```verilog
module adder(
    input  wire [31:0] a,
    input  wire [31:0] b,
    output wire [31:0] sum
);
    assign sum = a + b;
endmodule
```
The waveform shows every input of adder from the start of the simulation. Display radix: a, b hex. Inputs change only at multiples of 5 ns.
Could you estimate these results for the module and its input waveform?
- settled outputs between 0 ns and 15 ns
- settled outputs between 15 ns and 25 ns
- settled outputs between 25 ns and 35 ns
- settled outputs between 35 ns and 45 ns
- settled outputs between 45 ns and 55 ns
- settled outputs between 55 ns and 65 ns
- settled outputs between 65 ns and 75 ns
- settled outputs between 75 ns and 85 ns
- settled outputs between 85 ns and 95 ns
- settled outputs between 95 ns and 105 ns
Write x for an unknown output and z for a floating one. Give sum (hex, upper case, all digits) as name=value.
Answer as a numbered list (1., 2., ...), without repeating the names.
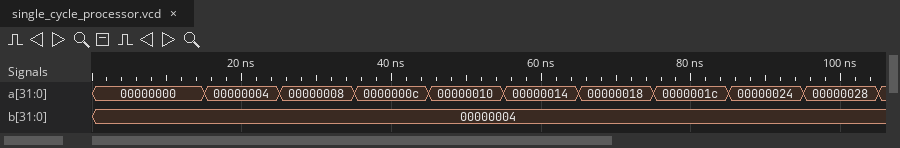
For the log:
1. sum=00000004
2. sum=00000008
3. sum=0000000C
4. sum=00000010
5. sum=00000014
6. sum=00000018
7. sum=0000001C
8. sum=00000020
9. sum=00000028
10. sum=0000002C
